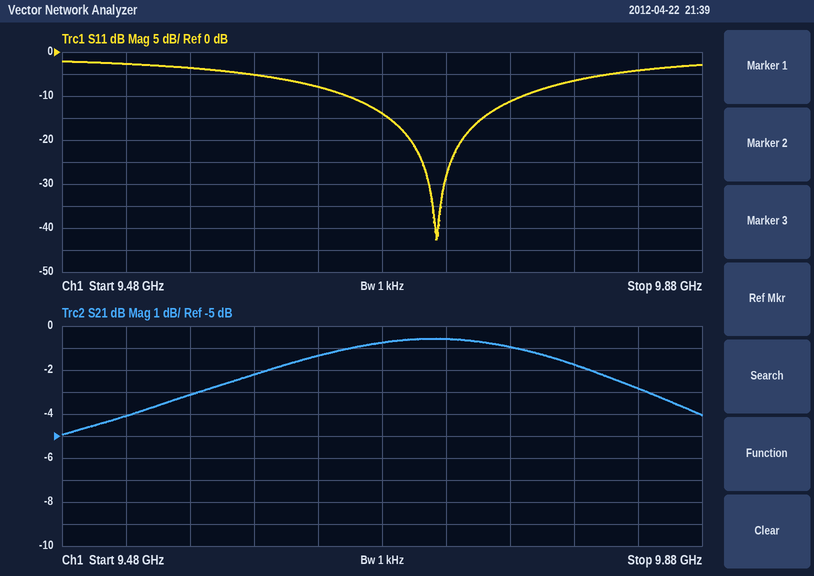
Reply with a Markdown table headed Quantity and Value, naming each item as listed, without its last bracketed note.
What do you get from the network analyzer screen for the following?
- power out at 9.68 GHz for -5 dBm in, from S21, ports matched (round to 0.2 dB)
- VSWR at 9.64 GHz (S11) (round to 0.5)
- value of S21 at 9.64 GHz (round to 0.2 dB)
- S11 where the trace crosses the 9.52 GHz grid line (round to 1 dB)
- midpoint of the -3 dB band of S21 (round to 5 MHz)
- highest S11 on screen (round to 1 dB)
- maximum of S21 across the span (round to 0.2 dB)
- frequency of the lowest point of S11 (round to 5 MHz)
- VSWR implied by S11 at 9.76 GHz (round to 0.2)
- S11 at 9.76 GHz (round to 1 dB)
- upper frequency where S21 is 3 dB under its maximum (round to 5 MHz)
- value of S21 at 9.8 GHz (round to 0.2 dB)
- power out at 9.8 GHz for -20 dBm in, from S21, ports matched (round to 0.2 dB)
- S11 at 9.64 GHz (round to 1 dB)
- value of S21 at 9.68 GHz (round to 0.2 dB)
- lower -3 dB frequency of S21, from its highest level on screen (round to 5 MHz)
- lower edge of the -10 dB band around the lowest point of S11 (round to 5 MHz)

| Quantity | Value |
|---|---|
| power out at 9.68 GHz for -5 dBm in, from S21, ports matched | -5.8 dBm |
| VSWR at 9.64 GHz (S11) | 2.5 |
| value of S21 at 9.64 GHz | -1.4 dB |
| S11 where the trace crosses the 9.52 GHz grid line | -3 dB |
| midpoint of the -3 dB band of S21 | 9.705 GHz |
| highest S11 on screen | -2 dB |
| maximum of S21 across the span | -0.6 dB |
| frequency of the lowest point of S11 | 9.715 GHz |
| VSWR implied by S11 at 9.76 GHz | 1.8 |
| S11 at 9.76 GHz | -11 dB |
| upper frequency where S21 is 3 dB under its maximum | 9.865 GHz |
| value of S21 at 9.8 GHz | -1.8 dB |
| power out at 9.8 GHz for -20 dBm in, from S21, ports matched | -21.8 dBm |
| S11 at 9.64 GHz | -8 dB |
| value of S21 at 9.68 GHz | -0.8 dB |
| lower -3 dB frequency of S21, from its highest level on screen | 9.540 GHz |
| lower edge of the -10 dB band around the lowest point of S11 | 9.660 GHz |
